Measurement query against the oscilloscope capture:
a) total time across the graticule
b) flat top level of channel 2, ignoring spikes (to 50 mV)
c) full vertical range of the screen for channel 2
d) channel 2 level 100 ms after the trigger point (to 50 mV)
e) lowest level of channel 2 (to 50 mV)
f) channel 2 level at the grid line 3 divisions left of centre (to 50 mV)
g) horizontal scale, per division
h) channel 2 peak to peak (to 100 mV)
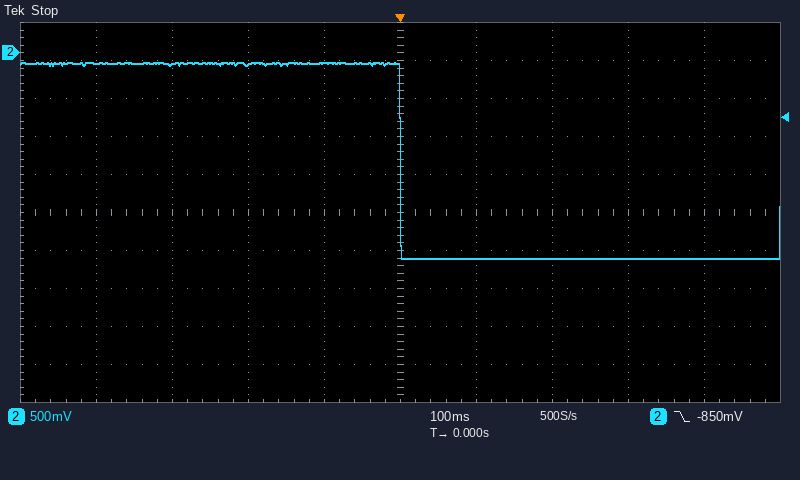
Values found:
1 s
-150 mV
5 V
-2.70 V
-2.70 V
-150 mV
100 ms
2.60 V
